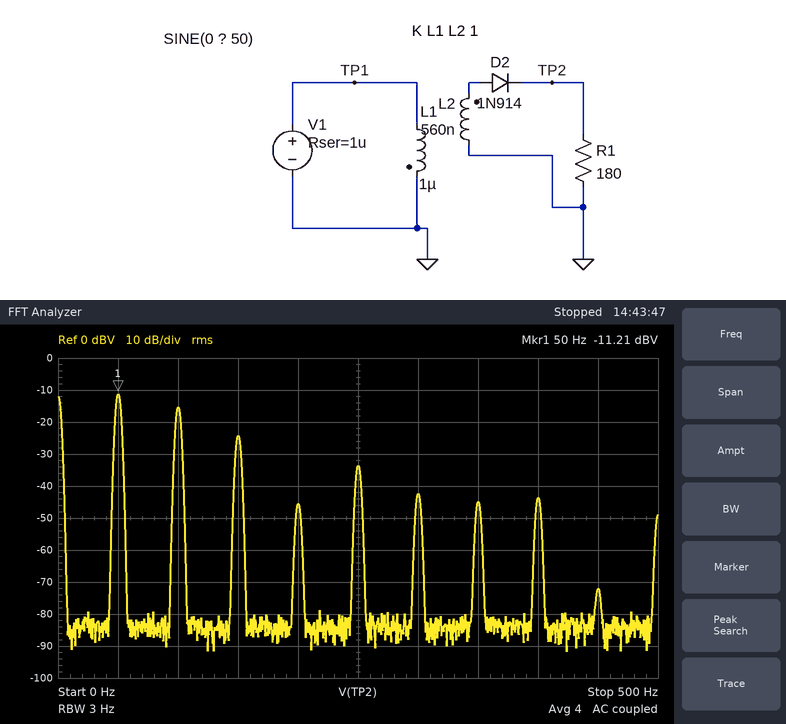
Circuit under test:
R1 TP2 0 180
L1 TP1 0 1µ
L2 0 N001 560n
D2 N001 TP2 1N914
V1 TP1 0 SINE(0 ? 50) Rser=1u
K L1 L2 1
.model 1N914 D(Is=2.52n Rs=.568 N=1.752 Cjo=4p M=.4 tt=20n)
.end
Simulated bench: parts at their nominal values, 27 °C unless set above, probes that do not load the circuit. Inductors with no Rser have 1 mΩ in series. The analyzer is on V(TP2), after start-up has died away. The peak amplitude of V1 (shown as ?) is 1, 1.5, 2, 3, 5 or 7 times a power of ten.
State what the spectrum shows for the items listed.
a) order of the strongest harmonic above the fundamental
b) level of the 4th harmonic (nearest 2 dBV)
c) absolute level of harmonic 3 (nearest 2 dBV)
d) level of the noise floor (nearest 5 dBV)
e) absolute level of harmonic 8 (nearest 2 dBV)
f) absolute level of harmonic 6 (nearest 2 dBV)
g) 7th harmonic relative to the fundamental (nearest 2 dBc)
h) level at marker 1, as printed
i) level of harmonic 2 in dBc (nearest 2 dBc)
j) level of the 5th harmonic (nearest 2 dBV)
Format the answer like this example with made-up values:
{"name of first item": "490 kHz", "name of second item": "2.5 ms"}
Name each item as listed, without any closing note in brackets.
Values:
{"order of the strongest harmonic above the fundamental": "2", "level of the 4th harmonic": "-46 dBV", "absolute level of harmonic 3": "-24 dBV", "level of the noise floor": "-85 dBV", "absolute level of harmonic 8": "-44 dBV", "absolute level of harmonic 6": "-42 dBV", "7th harmonic relative to the fundamental": "-34 dBc", "level at marker 1, as printed": "-11.21 dBV", "level of harmonic 2 in dBc": "-4 dBc", "level of the 5th harmonic": "-34 dBV"}
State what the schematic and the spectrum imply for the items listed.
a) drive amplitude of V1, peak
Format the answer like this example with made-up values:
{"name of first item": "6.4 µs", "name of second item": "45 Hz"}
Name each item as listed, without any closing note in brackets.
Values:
{"drive amplitude of V1, peak": "7 V"}
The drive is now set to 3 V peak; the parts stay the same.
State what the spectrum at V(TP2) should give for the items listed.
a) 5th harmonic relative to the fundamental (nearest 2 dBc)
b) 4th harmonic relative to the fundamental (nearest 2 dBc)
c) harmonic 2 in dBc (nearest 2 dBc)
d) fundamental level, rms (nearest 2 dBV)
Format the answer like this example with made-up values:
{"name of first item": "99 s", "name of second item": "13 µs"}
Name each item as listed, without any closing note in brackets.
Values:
{"5th harmonic relative to the fundamental": "-18 dBc", "4th harmonic relative to the fundamental": "-10 dBc", "harmonic 2 in dBc": "-2 dBc", "fundamental level, rms": "-32 dBV"}
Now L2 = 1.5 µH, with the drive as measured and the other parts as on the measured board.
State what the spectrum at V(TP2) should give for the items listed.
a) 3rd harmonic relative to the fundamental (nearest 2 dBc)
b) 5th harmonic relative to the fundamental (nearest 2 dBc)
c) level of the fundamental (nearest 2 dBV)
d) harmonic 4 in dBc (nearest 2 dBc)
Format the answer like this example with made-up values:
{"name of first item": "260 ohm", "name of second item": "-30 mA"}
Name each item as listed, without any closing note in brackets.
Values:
{"3rd harmonic relative to the fundamental": "-18 dBc", "5th harmonic relative to the fundamental": "-24 dBc", "level of the fundamental": "-4 dBV", "harmonic 4 in dBc": "-24 dBc"}
